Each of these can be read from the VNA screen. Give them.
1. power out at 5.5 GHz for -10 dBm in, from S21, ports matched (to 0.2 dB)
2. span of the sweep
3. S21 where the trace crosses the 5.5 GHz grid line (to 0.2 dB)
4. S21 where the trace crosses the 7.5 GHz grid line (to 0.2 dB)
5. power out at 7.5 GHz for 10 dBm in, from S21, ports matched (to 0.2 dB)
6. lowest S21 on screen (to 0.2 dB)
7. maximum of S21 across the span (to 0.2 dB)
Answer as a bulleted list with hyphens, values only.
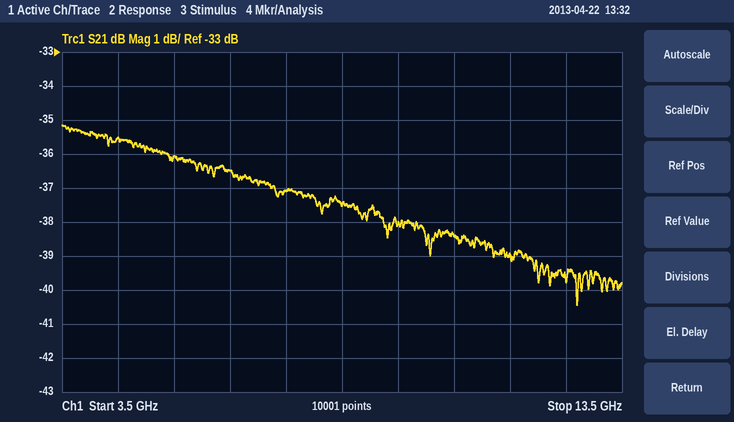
- -46.0 dBm
- 10 GHz
- -36.0 dB
- -37.0 dB
- -27.0 dBm
- -40.4 dB
- -35.2 dB
